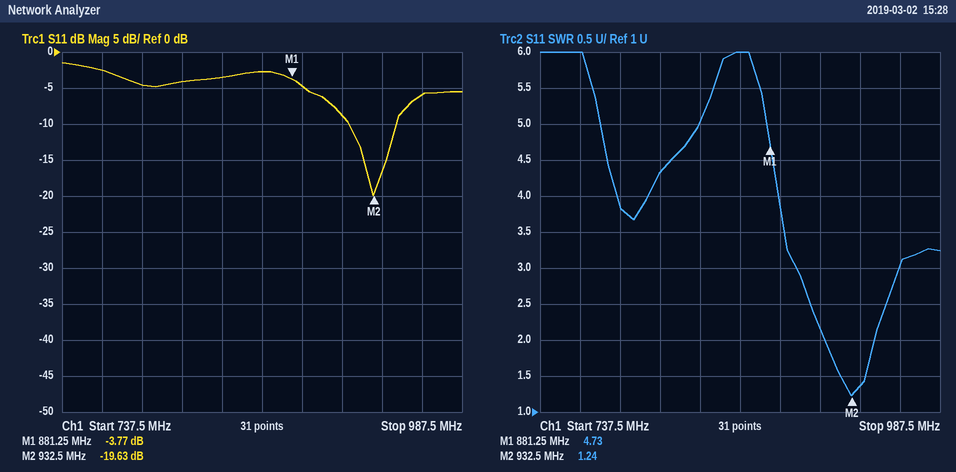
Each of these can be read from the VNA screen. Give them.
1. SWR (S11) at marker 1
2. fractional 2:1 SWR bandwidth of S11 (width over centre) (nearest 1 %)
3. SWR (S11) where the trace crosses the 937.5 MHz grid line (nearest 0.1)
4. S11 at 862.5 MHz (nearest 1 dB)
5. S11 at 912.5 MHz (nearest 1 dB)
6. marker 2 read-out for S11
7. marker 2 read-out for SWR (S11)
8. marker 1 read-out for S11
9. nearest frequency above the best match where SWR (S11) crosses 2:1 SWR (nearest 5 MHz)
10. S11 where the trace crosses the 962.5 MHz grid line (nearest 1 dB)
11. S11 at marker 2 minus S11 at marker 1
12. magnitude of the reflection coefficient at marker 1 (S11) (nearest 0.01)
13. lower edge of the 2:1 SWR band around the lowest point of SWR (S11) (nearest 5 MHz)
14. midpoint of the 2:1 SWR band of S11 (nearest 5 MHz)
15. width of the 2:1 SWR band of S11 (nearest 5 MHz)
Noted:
4.73
3 %
1.4
-3 dB
-9 dB
-19.63 dB
1.24
-3.77 dB
945 MHz
-6 dB
-15.86 dB
0.65
915 MHz
930 MHz
30 MHz
